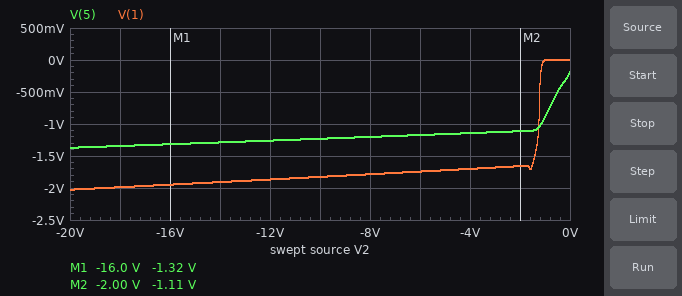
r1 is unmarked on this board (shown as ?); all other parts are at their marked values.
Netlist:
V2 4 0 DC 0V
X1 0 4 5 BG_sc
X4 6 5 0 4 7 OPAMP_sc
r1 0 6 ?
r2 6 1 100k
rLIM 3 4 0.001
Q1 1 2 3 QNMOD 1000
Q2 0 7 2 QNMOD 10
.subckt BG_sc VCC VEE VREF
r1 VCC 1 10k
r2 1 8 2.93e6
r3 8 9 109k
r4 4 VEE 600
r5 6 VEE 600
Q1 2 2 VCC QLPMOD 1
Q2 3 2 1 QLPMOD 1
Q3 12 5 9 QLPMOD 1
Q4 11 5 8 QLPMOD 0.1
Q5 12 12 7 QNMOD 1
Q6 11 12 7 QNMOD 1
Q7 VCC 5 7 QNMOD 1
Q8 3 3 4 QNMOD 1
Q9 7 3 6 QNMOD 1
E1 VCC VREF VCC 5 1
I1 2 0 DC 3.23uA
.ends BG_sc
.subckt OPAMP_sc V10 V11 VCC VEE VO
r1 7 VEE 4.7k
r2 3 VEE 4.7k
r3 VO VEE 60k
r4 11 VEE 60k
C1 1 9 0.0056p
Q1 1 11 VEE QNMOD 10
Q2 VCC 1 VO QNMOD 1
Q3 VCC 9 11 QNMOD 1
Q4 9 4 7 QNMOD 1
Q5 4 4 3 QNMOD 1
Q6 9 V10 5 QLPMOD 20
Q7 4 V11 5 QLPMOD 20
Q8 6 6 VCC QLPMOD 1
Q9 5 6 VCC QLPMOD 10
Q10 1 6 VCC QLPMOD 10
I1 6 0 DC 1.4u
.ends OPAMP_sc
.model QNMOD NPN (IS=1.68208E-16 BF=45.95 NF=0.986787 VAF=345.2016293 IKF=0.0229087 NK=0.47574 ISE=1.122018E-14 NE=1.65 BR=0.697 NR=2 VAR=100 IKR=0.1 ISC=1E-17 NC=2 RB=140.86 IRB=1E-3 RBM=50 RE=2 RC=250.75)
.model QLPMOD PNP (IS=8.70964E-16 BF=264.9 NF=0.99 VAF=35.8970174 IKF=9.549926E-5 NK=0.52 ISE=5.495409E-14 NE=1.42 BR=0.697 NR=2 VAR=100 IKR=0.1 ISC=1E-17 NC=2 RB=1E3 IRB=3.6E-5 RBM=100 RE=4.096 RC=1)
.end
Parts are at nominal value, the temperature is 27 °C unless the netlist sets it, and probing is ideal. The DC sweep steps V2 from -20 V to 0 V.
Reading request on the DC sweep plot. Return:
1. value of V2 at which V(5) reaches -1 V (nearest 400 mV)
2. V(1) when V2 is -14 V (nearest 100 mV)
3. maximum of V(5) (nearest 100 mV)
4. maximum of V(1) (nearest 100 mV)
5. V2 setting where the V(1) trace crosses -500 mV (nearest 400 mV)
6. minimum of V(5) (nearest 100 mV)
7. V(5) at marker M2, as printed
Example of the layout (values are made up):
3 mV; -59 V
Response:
-1.2 V; -1.9 V; -200 mV; 0 V; -1.2 V; -1.4 V; -1.11 V
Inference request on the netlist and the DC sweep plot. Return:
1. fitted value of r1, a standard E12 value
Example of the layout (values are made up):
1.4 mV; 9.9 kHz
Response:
220 kΩ
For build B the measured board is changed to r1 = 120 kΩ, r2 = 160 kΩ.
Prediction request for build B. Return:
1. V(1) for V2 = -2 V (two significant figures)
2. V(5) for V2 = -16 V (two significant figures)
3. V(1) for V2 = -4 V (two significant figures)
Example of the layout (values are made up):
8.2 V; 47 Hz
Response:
-2.2 V; -1.3 V; -2.7 V
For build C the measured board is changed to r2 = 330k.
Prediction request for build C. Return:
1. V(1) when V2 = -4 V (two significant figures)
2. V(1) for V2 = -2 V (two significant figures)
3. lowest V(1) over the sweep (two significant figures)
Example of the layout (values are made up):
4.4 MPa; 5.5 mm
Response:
-3.0 V; -2.2 V; -3.5 V
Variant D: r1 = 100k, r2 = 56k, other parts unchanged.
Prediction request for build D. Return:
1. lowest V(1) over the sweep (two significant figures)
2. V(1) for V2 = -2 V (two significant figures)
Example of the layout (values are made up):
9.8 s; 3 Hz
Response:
-2.2 V; -1.8 V
